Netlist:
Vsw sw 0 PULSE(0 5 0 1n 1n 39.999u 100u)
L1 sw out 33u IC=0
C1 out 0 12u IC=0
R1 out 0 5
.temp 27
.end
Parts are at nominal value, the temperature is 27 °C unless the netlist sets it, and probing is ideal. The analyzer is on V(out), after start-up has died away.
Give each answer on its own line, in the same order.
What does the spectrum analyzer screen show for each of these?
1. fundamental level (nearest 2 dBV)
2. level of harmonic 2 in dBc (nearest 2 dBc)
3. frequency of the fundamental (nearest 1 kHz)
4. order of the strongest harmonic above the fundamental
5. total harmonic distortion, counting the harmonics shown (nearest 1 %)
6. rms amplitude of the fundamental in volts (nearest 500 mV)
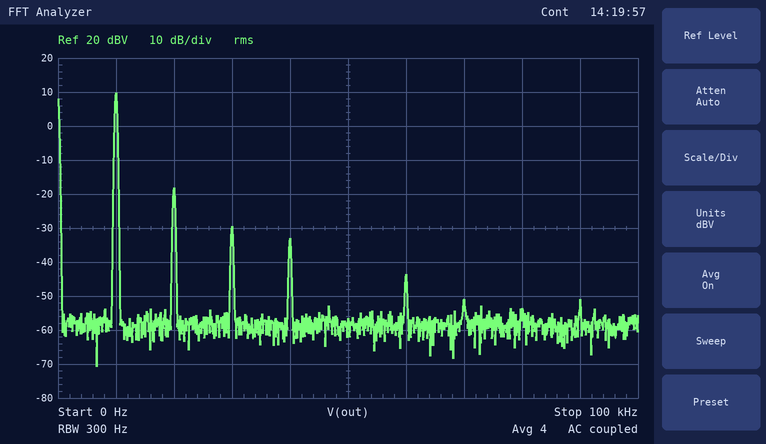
10 dBV
-28 dBc
10 kHz
2
4 %
3.0 V
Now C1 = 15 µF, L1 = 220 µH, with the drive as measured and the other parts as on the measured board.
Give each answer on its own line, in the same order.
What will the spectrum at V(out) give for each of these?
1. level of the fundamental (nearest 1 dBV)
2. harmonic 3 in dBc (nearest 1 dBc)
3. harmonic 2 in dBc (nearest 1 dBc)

-15 dBV
-33 dBc
-23 dBc
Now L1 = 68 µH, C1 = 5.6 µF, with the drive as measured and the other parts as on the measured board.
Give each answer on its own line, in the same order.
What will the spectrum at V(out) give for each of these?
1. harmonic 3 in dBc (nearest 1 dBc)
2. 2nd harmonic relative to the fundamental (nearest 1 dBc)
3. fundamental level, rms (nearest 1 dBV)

-36 dBc
-25 dBc
7 dBV
